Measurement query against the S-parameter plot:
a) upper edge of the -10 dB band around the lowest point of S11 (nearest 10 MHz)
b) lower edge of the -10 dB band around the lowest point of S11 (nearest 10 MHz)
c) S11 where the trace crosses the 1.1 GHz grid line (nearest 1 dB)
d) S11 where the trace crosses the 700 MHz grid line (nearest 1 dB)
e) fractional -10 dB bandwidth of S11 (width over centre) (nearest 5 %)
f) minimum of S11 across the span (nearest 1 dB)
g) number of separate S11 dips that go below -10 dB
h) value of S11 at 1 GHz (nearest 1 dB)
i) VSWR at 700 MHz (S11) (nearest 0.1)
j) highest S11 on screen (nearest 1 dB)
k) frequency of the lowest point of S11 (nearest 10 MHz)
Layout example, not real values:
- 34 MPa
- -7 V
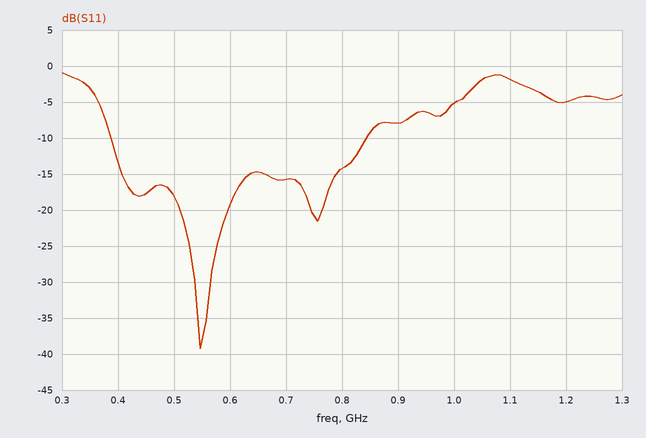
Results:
- 840 MHz
- 390 MHz
- -2 dB
- -16 dB
- 75 %
- -39 dB
- 2
- -5 dB
- 1.4
- -1 dB
- 550 MHz
